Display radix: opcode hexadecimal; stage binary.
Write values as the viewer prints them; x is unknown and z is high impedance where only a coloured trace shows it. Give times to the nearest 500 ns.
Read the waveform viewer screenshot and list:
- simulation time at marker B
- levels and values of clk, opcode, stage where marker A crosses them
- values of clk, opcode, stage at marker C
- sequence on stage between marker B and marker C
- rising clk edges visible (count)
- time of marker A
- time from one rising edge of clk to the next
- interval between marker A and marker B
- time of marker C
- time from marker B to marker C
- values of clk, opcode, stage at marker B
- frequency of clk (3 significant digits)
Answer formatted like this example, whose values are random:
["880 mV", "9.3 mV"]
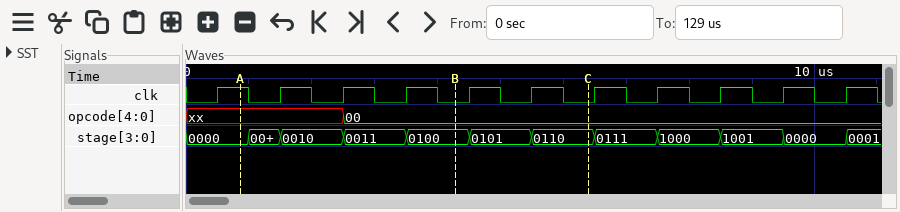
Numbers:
["4500 ns", "clk=1, opcode=xx, stage=0000", "clk=0, opcode=00, stage=0110", "0100, 0101, 0110", "11", "1000 ns", "1000 ns", "3500 ns", "6500 ns", "2000 ns", "clk=0, opcode=00, stage=0100", "1.00 MHz"]
